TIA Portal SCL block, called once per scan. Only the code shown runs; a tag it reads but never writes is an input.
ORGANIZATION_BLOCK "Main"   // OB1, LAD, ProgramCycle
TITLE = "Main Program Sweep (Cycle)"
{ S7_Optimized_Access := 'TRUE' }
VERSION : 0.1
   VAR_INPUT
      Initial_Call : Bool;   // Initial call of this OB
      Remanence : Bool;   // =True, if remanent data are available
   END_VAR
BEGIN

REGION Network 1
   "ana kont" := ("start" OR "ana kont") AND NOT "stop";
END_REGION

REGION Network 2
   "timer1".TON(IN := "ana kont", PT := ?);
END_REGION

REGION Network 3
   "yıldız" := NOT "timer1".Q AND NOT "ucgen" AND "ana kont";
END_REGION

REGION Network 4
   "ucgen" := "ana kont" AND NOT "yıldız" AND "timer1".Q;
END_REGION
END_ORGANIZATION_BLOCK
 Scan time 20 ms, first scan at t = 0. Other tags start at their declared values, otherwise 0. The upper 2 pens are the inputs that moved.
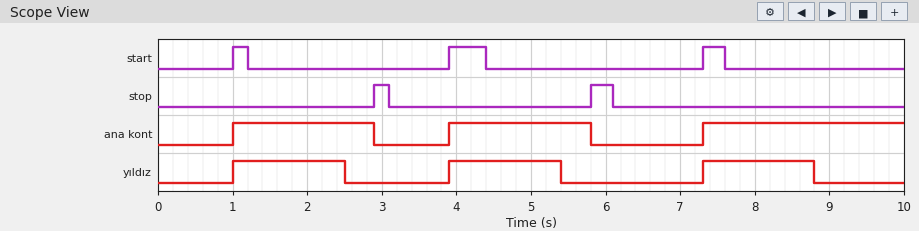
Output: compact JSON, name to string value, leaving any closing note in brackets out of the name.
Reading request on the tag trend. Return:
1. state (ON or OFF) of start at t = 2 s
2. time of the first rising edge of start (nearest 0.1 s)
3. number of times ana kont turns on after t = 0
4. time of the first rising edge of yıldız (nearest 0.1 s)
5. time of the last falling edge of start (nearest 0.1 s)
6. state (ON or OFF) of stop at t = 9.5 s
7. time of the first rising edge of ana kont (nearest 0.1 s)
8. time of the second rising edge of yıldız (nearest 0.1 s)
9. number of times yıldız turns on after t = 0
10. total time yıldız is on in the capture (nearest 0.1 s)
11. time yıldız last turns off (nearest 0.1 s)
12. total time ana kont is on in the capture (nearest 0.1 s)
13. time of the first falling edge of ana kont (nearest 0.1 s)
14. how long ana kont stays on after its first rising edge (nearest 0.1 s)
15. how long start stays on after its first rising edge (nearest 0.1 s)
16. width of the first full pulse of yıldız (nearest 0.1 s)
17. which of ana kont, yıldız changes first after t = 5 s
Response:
{"state (ON or OFF) of start at t = 2 s": "OFF", "time of the first rising edge of start": "1.0 s", "number of times ana kont turns on after t = 0": "3", "time of the first rising edge of yıldız": "1.0 s", "time of the last falling edge of start": "7.6 s", "state (ON or OFF) of stop at t = 9.5 s": "OFF", "time of the first rising edge of ana kont": "1.0 s", "time of the second rising edge of yıldız": "3.9 s", "number of times yıldız turns on after t = 0": "3", "total time yıldız is on in the capture": "4.5 s", "time yıldız last turns off": "8.8 s", "total time ana kont is on in the capture": "6.5 s", "time of the first falling edge of ana kont": "2.9 s", "how long ana kont stays on after its first rising edge": "1.9 s", "how long start stays on after its first rising edge": "0.2 s", "width of the first full pulse of yıldız": "1.5 s", "which of ana kont, yıldız changes first after t = 5 s": "yıldız"}
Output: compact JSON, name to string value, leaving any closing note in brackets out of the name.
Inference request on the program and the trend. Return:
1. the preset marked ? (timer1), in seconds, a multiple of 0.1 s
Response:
{"the preset marked ? (timer1), in seconds, a multiple of 0.1 s": "1.5 s"}
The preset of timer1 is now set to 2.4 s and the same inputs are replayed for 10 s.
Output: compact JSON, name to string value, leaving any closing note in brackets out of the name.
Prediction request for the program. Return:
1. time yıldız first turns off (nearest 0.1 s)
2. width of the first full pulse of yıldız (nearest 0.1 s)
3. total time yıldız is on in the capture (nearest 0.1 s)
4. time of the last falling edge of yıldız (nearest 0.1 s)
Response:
{"time yıldız first turns off": "2.9 s", "width of the first full pulse of yıldız": "1.9 s", "total time yıldız is on in the capture": "6.2 s", "time of the last falling edge of yıldız": "9.7 s"}
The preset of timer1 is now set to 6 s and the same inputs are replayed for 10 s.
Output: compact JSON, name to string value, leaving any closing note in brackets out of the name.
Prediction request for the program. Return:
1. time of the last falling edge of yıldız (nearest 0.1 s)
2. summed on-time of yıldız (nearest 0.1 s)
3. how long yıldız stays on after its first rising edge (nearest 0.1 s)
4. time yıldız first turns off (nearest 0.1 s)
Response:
{"time of the last falling edge of yıldız": "5.8 s", "summed on-time of yıldız": "6.5 s", "how long yıldız stays on after its first rising edge": "1.9 s", "time yıldız first turns off": "2.9 s"}
